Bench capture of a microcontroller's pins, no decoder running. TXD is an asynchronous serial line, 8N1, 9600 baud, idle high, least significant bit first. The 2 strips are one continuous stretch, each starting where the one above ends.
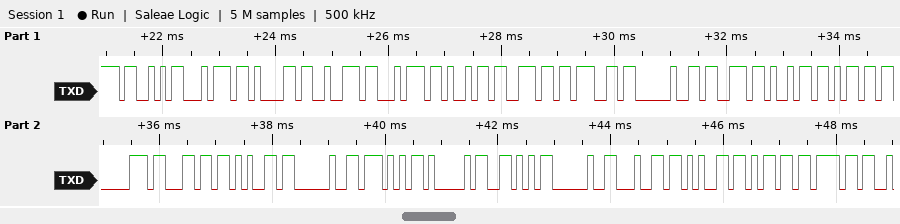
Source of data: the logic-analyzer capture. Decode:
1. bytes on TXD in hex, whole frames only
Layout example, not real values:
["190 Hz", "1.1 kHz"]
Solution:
["53 74 61 72 74 69 6E 67 20 73 69 6D 70 6C 65 20 57 41 56 20 64 65 6D 6F"]
